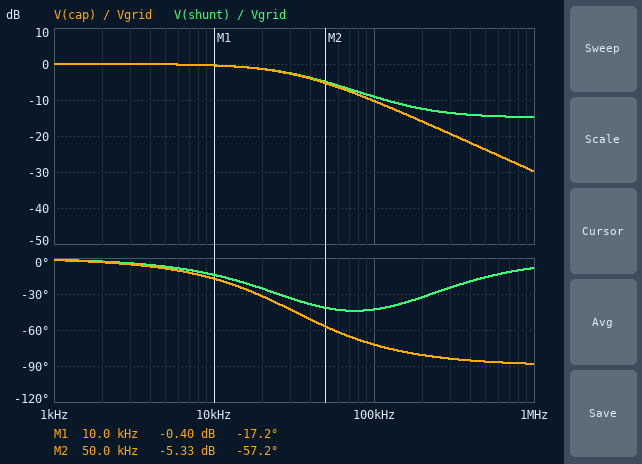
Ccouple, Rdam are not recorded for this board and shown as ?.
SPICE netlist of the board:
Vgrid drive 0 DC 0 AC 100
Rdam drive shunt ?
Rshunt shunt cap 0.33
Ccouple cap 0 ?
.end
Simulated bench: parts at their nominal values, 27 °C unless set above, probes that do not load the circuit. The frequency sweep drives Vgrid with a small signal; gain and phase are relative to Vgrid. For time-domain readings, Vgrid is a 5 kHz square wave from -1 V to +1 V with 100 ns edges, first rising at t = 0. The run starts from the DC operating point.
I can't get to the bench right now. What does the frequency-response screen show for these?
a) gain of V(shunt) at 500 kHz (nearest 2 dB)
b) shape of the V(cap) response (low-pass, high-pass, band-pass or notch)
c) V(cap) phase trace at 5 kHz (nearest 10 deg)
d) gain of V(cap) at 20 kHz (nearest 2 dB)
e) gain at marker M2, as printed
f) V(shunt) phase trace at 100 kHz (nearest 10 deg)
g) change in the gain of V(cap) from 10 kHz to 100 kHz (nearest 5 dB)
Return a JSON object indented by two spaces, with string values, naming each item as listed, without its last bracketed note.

{
  "gain of V(shunt) at 500 kHz": "-14 dB",
  "shape of the V(cap) response": "low-pass",
  "V(cap) phase trace at 5 kHz": "-10 deg",
  "gain of V(cap) at 20 kHz": "-2 dB",
  "gain at marker M2, as printed": "-5.33 dB",
  "V(shunt) phase trace at 100 kHz": "-40 deg",
  "change in the gain of V(cap) from 10 kHz to 100 kHz": "-10 dB"
}
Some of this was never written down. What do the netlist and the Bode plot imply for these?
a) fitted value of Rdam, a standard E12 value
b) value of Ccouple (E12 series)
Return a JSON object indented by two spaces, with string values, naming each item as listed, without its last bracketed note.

{
  "fitted value of Rdam, a standard E12 value": "1.5 Ω",
  "value of Ccouple": "2.7 µF"
}
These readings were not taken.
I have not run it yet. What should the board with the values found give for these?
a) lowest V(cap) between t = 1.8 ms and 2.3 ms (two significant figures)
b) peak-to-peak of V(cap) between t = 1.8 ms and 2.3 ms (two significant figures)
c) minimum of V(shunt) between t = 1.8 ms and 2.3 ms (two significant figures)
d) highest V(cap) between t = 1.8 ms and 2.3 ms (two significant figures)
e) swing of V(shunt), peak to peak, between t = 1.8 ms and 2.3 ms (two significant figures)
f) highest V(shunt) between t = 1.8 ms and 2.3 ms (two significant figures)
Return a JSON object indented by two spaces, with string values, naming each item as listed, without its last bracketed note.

{
  "lowest V(cap) between t = 1.8 ms and 2.3 ms": "-1.0 V",
  "peak-to-peak of V(cap) between t = 1.8 ms and 2.3 ms": "2.0 V",
  "minimum of V(shunt) between t = 1.8 ms and 2.3 ms": "-1.0 V",
  "highest V(cap) between t = 1.8 ms and 2.3 ms": "1.0 V",
  "swing of V(shunt), peak to peak, between t = 1.8 ms and 2.3 ms": "2.0 V",
  "highest V(shunt) between t = 1.8 ms and 2.3 ms": "1.0 V"
}
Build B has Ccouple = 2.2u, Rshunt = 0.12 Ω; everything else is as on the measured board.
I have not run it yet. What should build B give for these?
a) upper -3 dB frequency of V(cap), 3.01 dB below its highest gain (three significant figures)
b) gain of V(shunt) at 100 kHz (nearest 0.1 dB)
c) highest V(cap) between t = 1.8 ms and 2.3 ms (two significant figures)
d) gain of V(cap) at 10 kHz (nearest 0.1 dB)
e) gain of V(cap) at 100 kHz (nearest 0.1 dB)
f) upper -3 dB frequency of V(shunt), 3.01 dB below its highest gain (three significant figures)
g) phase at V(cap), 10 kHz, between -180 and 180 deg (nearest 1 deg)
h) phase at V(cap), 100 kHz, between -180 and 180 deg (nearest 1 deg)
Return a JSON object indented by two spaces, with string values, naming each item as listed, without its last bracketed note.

{
  "upper -3 dB frequency of V(cap), 3.01 dB below its highest gain": "44.7 kHz",
  "gain of V(shunt) at 100 kHz": "-7.7 dB",
  "highest V(cap) between t = 1.8 ms and 2.3 ms": "1.0 V",
  "gain of V(cap) at 10 kHz": "-0.2 dB",
  "gain of V(cap) at 100 kHz": "-7.8 dB",
  "upper -3 dB frequency of V(shunt), 3.01 dB below its highest gain": "44.9 kHz",
  "phase at V(cap), 10 kHz, between -180 and 180 deg": "-13 deg",
  "phase at V(cap), 100 kHz, between -180 and 180 deg": "-66 deg"
}
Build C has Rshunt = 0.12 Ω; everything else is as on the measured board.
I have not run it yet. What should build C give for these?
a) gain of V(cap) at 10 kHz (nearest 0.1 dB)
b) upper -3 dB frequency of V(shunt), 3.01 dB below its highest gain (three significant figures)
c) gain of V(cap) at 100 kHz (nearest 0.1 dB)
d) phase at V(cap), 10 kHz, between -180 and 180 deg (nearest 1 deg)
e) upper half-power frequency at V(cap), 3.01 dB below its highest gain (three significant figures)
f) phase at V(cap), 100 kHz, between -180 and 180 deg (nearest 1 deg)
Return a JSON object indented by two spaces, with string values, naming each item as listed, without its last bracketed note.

{
  "gain of V(cap) at 10 kHz": "-0.3 dB",
  "upper -3 dB frequency of V(shunt), 3.01 dB below its highest gain": "36.6 kHz",
  "gain of V(cap) at 100 kHz": "-9.3 dB",
  "phase at V(cap), 10 kHz, between -180 and 180 deg": "-15 deg",
  "upper half-power frequency at V(cap), 3.01 dB below its highest gain": "36.4 kHz",
  "phase at V(cap), 100 kHz, between -180 and 180 deg": "-70 deg"
}
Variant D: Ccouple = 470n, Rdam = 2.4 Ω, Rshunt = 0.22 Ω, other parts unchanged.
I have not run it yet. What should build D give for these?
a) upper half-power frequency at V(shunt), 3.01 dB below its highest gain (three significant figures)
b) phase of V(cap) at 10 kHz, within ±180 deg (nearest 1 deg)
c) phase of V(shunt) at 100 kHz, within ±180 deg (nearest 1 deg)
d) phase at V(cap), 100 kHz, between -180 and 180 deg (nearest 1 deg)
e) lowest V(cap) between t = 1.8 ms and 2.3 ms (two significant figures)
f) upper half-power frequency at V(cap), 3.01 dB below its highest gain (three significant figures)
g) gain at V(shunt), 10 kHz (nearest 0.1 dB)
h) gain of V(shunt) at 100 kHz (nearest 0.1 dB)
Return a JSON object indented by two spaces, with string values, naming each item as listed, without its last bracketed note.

{
  "upper half-power frequency at V(shunt), 3.01 dB below its highest gain": "130 kHz",
  "phase of V(cap) at 10 kHz, within ±180 deg": "-4 deg",
  "phase of V(shunt) at 100 kHz, within ±180 deg": "-34 deg",
  "phase at V(cap), 100 kHz, between -180 and 180 deg": "-38 deg",
  "lowest V(cap) between t = 1.8 ms and 2.3 ms": "-1.0 V",
  "upper half-power frequency at V(cap), 3.01 dB below its highest gain": "129 kHz",
  "gain at V(shunt), 10 kHz": "0 dB",
  "gain of V(shunt) at 100 kHz": "-2.0 dB"
}
